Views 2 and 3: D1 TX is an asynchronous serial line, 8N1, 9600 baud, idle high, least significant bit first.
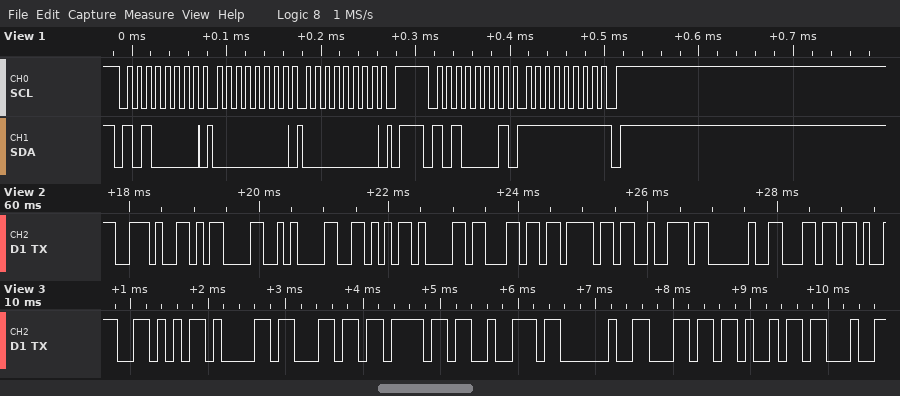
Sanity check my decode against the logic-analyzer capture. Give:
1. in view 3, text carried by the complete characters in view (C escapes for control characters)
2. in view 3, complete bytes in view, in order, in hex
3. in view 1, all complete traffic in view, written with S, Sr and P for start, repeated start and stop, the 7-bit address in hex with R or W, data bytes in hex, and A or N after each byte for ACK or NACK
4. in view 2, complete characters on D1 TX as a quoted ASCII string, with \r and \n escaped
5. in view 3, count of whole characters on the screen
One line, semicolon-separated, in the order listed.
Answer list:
"Valor li"; 56 61 6C 6F 72 20 6C 69; S 50W A 00 A 00 A P S 50R A FF N P; ".\r\nValor l"; 8
